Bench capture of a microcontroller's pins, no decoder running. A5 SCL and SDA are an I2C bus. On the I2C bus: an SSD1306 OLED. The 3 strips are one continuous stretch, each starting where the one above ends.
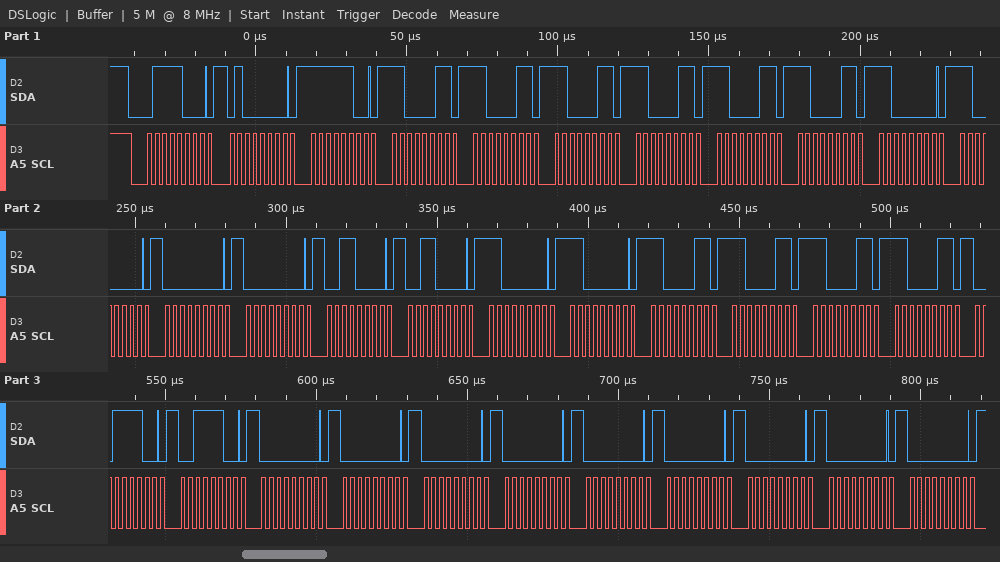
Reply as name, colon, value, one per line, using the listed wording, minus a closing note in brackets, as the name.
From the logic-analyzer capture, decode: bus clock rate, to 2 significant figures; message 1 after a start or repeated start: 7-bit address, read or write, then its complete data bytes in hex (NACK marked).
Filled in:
bus clock rate, to 2 significant figures: 400 kHz
message 1 after a start or repeated start: 7-bit address, read or write, then its complete data bytes in hex: 0x3C write: 40 FC C3 C3 C3 C3 C3 C3 C0 C0 00 00 30 30 C0 C0 C3 C3 C3 C3 3C 3C 00 00 00 00 00 00 00 00 00
